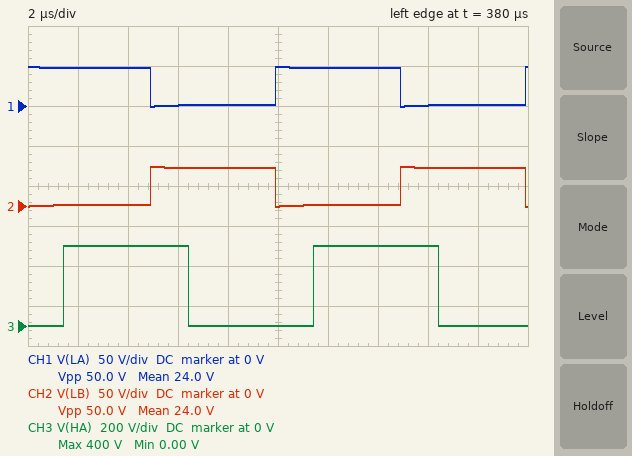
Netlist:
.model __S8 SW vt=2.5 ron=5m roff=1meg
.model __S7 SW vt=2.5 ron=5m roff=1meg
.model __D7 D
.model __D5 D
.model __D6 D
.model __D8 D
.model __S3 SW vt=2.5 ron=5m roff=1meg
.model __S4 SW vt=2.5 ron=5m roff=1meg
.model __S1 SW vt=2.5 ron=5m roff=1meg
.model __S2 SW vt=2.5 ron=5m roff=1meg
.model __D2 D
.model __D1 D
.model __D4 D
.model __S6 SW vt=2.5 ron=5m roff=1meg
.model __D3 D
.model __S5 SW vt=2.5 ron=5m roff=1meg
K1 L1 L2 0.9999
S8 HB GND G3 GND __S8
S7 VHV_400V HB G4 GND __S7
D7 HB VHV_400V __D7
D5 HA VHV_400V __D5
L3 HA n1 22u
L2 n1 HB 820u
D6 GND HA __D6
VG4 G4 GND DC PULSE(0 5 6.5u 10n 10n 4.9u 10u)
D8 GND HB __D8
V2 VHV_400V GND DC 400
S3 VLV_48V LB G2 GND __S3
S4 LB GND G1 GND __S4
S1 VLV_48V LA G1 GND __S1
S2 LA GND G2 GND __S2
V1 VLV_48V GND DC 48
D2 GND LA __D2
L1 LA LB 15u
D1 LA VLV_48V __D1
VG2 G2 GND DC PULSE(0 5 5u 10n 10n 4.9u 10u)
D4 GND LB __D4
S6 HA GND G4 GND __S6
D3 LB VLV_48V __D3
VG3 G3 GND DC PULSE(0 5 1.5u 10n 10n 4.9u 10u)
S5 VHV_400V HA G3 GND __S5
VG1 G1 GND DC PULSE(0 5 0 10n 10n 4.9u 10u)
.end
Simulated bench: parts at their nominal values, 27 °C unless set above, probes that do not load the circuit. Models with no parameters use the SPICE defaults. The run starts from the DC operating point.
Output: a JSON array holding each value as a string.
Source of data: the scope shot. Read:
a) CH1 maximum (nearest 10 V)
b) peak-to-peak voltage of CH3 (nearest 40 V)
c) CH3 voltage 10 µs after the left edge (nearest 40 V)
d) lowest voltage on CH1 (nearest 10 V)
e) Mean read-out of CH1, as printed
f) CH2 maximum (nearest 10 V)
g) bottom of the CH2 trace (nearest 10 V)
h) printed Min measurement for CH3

["50 V", "400 V", "0 V", "0 V", "24.0 V", "50 V", "0 V", "0.00 V"]
